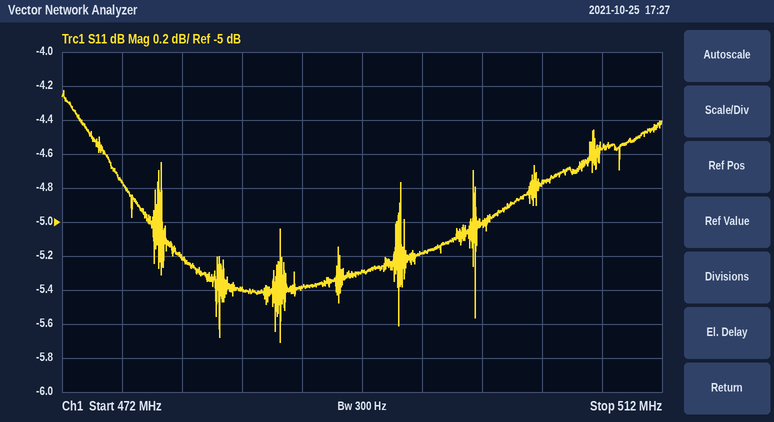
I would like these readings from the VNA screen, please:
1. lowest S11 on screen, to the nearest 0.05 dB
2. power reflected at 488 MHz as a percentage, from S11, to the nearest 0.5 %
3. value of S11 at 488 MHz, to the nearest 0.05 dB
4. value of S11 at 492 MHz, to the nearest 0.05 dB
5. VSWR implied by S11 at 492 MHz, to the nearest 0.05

-5.70 dB
29.0 %
-5.40 dB
-5.30 dB
3.40
